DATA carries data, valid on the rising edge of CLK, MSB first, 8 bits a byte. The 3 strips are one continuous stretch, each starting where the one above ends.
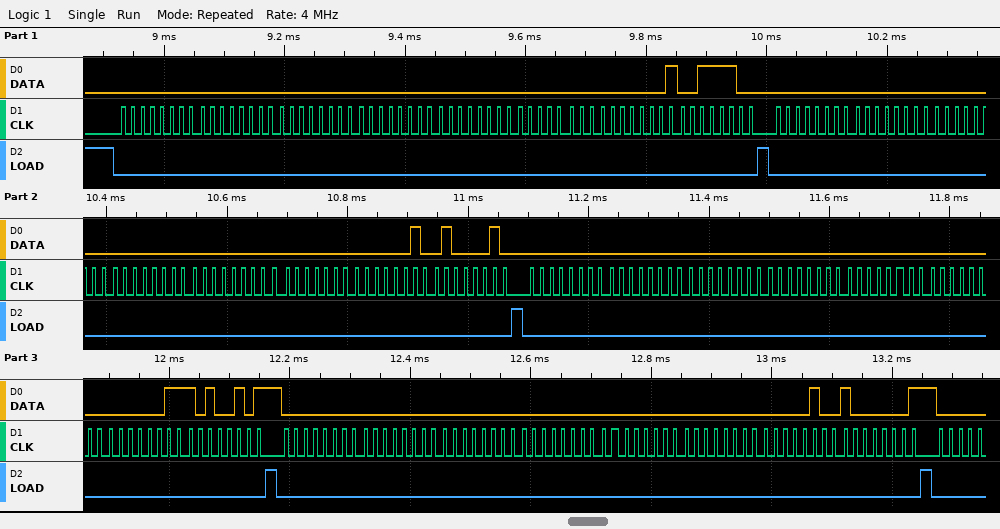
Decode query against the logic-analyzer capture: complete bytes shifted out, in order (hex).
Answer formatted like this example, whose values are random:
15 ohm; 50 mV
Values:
00 00 00 00 00 00 01 3C 00 00 00 00 00 00 02 42 00 00 00 00 00 00 03 A5 00 00 00 00 00 00 04 81
